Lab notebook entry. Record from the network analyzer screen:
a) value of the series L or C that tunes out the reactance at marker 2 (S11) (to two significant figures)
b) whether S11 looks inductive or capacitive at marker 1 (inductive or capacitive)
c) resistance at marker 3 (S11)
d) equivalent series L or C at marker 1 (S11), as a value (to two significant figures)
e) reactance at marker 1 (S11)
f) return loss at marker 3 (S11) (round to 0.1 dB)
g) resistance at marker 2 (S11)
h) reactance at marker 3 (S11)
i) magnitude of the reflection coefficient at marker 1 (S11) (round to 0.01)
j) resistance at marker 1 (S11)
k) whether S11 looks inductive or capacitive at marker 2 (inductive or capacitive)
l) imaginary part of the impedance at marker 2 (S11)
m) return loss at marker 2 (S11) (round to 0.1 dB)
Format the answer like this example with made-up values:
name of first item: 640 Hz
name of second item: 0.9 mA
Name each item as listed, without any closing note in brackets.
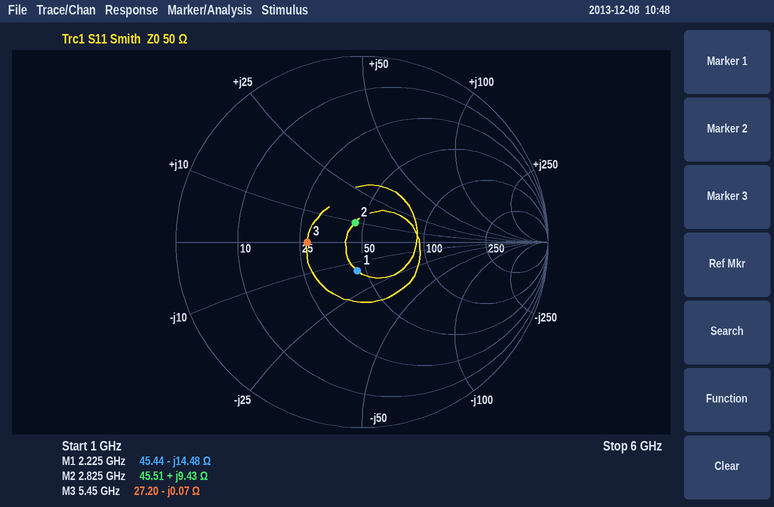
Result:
value of the series L or C that tunes out the reactance at marker 2 (S11): 6.0 pF
whether S11 looks inductive or capacitive at marker 1: capacitive
resistance at marker 3: 27.20 Ω
equivalent series L or C at marker 1 (S11), as a value: 4.9 pF
reactance at marker 1: -14.48 Ω
return loss at marker 3 (S11): 10.6 dB
resistance at marker 2: 45.51 Ω
reactance at marker 3: -0.07 Ω
magnitude of the reflection coefficient at marker 1 (S11): 0.16
resistance at marker 1: 45.44 Ω
whether S11 looks inductive or capacitive at marker 2: inductive
imaginary part of the impedance at marker 2: +9.43 Ω
return loss at marker 2 (S11): 19.3 dB
